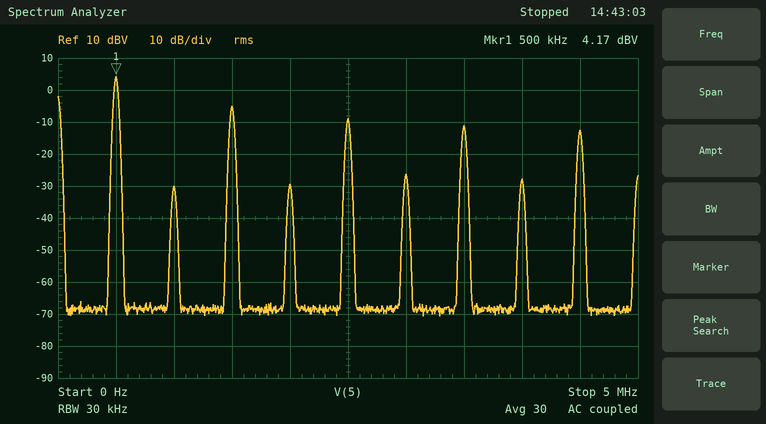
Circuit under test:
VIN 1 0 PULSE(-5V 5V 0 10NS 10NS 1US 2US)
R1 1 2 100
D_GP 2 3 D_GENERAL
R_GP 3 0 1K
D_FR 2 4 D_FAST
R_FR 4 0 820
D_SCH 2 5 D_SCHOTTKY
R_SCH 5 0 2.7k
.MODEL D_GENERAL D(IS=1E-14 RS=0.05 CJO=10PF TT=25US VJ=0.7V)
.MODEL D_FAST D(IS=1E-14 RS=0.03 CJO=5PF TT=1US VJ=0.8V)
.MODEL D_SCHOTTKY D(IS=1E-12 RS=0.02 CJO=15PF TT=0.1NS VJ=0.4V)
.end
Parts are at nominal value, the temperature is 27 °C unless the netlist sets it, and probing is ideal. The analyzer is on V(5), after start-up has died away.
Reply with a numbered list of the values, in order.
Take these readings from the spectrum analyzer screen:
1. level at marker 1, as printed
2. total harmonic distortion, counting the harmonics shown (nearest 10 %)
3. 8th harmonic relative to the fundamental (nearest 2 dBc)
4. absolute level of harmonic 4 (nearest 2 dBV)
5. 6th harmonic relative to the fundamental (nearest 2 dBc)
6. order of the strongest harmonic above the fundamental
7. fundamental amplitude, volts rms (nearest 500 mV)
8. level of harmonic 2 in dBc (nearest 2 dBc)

1. 4.17 dBV
2. 50 %
3. -32 dBc
4. -30 dBV
5. -30 dBc
6. 3
7. 1.5 V
8. -34 dBc
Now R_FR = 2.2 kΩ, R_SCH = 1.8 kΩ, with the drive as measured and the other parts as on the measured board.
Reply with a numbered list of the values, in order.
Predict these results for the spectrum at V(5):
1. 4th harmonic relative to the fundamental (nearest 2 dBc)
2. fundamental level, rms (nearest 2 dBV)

1. -38 dBc
2. 4 dBV
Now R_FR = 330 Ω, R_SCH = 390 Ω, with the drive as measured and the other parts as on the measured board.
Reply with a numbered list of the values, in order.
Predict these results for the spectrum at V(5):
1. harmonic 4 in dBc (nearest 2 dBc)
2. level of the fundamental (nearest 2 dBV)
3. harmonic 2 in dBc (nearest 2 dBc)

1. -48 dBc
2. 2 dBV
3. -46 dBc
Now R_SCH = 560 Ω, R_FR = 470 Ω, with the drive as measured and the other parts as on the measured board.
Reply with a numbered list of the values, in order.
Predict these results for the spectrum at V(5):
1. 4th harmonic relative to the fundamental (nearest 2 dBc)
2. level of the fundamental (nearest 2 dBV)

1. -50 dBc
2. 2 dBV
